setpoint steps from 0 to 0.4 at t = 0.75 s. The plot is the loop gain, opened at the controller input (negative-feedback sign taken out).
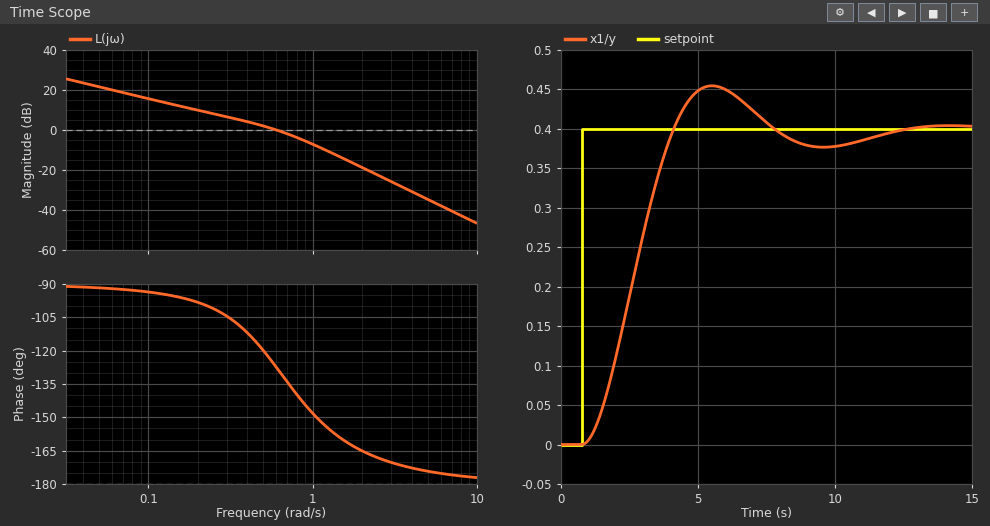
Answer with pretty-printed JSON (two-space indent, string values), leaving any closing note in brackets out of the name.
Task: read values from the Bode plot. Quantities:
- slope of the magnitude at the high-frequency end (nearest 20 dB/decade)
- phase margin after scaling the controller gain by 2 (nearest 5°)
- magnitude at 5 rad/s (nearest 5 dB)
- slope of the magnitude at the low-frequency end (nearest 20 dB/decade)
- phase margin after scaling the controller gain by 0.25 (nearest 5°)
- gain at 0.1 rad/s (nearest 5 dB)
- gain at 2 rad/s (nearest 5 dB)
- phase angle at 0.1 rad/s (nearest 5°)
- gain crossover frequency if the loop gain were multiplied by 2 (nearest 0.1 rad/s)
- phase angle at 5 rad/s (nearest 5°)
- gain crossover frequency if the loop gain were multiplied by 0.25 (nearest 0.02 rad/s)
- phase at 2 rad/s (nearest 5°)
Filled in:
{
  "slope of the magnitude at the high-frequency end": "-40 dB/decade",
  "phase margin after scaling the controller gain by 2": "35°",
  "magnitude at 5 rad/s": "-35 dB",
  "slope of the magnitude at the low-frequency end": "-20 dB/decade",
  "phase margin after scaling the controller gain by 0.25": "85°",
  "gain at 0.1 rad/s": "15 dB",
  "gain at 2 rad/s": "-20 dB",
  "phase angle at 0.1 rad/s": "-95°",
  "gain crossover frequency if the loop gain were multiplied by 2": "0.9 rad/s",
  "phase angle at 5 rad/s": "-175°",
  "gain crossover frequency if the loop gain were multiplied by 0.25": "0.16 rad/s",
  "phase at 2 rad/s": "-165°"
}
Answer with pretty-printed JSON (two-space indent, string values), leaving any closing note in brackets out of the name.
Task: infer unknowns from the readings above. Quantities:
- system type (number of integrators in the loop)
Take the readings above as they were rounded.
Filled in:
{
  "system type": "1"
}
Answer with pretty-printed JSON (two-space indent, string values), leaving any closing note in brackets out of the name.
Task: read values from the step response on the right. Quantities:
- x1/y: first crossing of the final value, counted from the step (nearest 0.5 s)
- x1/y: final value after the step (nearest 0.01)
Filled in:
{
  "x1/y: first crossing of the final value, counted from the step": "3.5 s",
  "x1/y: final value after the step": "0.40"
}
